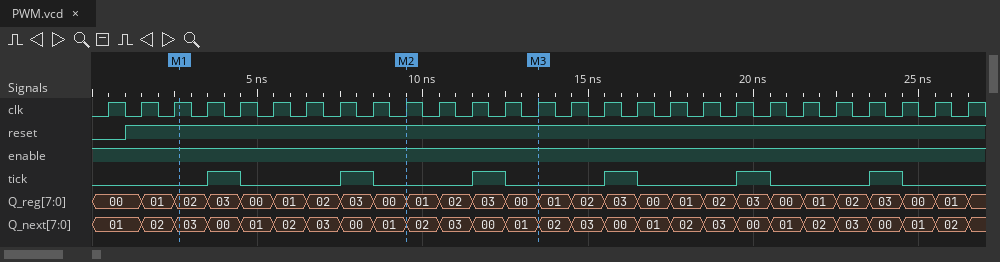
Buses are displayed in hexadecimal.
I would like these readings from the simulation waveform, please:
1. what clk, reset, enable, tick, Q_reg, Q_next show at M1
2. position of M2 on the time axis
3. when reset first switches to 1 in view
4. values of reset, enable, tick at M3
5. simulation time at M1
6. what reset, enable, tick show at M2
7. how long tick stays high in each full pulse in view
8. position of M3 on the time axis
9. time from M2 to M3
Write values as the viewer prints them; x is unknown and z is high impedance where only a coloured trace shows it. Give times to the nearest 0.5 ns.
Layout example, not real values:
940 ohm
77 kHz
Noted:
clk=1, reset=1, enable=1, tick=0, Q_reg=02, Q_next=03
9.5 ns
1 ns
reset=1, enable=1, tick=0
2.5 ns
reset=1, enable=1, tick=0
1 ns, 1 ns, 1 ns, 1 ns, 1 ns, 1 ns
13.5 ns
4 ns
